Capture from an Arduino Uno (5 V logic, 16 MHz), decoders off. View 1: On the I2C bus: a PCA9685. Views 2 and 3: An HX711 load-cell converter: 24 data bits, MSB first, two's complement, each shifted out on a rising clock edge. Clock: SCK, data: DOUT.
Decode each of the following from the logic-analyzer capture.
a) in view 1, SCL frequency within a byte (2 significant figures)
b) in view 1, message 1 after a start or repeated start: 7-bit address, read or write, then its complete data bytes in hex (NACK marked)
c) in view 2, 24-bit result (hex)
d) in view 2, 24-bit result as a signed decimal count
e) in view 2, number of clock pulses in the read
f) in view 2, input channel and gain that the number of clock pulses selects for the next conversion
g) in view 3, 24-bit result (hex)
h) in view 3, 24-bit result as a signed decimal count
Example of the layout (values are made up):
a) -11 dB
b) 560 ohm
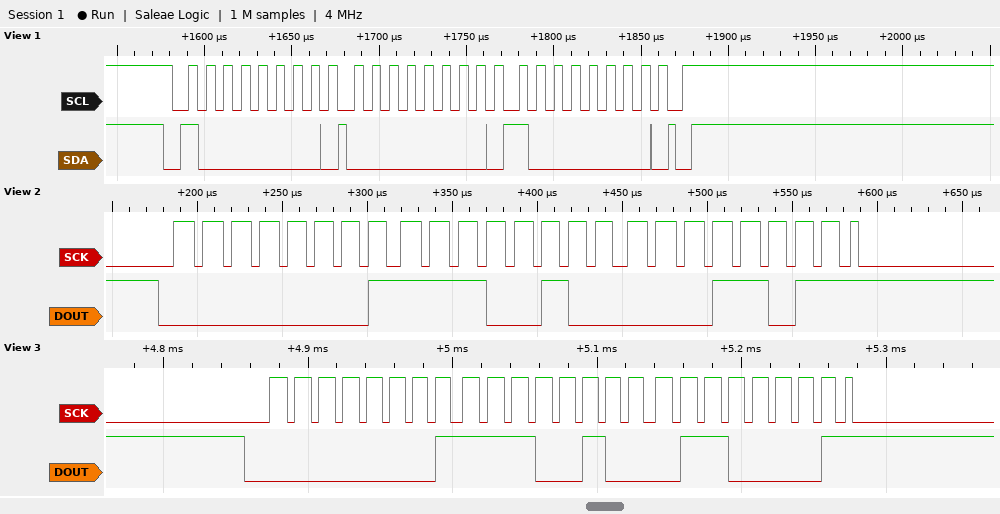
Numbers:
a) 100 kHz
b) 0x40 write: 00 80
c) 0x01E41B
d) 123931
e) 25
f) channel A, gain 128
g) 0x01E461
h) 124001
